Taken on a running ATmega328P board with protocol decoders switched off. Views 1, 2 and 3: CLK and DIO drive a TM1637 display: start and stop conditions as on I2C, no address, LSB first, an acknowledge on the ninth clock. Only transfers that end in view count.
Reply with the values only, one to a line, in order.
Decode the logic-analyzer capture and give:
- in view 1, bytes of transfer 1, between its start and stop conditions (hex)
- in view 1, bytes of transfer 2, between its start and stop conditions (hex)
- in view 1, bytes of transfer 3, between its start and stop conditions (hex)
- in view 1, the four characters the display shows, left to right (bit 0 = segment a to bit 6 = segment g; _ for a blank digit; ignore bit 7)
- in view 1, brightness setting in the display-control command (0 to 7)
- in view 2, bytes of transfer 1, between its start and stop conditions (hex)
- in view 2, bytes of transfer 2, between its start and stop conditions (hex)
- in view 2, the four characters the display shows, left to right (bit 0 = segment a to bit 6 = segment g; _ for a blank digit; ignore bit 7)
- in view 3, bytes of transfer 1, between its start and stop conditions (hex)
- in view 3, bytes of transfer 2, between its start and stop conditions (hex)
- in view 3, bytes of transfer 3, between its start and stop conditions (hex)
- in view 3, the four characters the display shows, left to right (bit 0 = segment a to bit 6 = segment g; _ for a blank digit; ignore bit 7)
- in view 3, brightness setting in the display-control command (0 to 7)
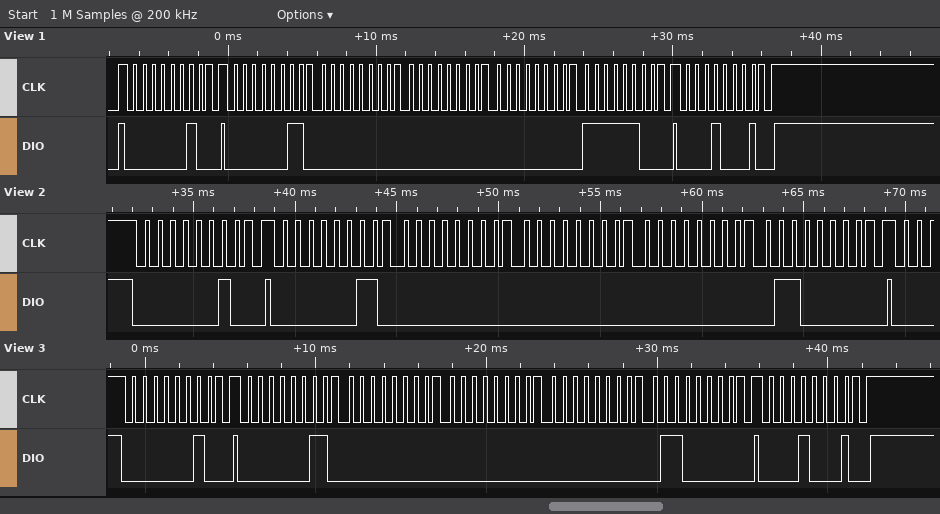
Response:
40
C0 00 00 00 3F
88
___0
0
40
C0 00 00 00 06
___1
40
C0 00 00 00 06
88
___1
0
